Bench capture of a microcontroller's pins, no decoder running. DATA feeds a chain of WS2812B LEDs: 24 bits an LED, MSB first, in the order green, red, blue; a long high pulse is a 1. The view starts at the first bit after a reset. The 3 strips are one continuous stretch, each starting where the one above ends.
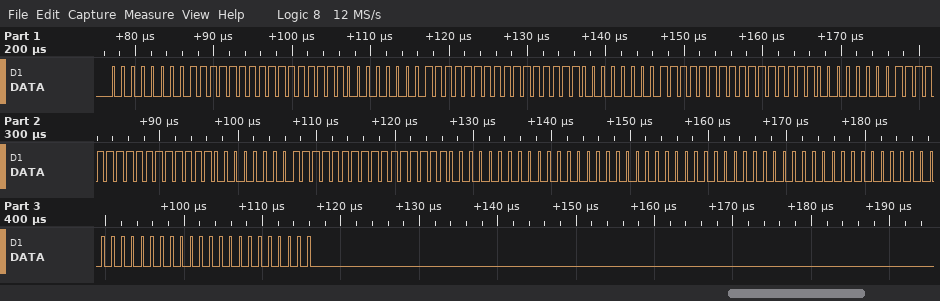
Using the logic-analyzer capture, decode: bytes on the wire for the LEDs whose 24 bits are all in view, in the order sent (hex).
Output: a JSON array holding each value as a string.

["00 FF FF 00 FF FF 00 FF FF 00 FF FF 00 FF FF 00 00 00 00 00 00 00 00 00"]
